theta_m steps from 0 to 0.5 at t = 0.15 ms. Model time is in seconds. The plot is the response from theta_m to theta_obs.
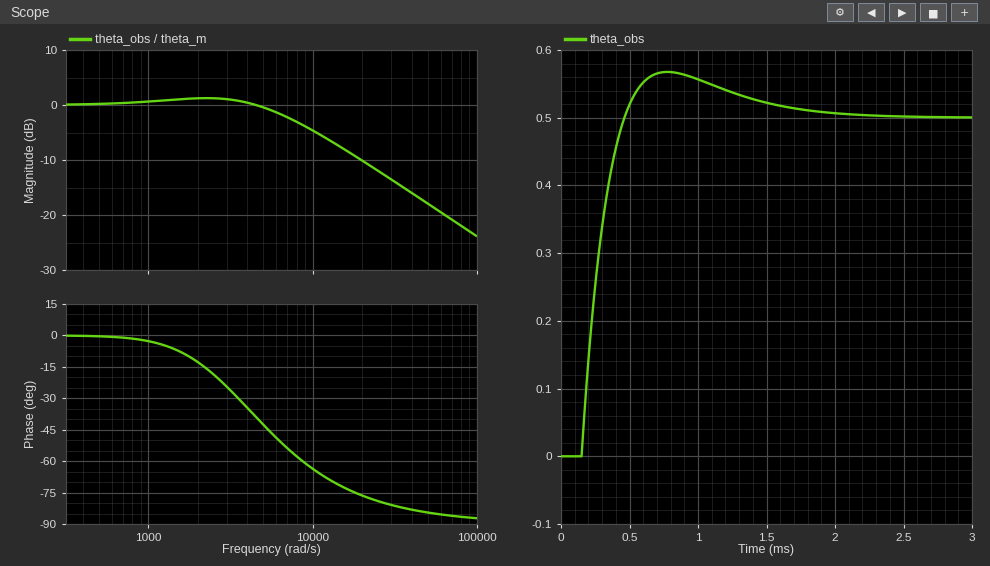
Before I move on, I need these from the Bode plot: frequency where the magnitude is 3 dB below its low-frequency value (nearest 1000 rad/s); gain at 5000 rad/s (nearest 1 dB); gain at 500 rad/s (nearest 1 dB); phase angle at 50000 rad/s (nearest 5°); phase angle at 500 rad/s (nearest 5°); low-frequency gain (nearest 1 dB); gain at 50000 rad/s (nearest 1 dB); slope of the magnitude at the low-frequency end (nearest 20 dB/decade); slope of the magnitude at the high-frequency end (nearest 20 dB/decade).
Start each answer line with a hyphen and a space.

- 8000 rad/s
- 0 dB
- 0 dB
- -85°
- 0°
- 0 dB
- -18 dB
- 0 dB/decade
- -20 dB/decade
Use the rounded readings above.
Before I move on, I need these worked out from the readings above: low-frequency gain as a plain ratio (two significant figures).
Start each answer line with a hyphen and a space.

- 1.0
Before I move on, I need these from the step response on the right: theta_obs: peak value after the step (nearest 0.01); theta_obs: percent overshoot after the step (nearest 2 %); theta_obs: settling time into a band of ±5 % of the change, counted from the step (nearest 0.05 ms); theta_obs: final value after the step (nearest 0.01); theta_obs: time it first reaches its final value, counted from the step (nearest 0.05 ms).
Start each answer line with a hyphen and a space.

- 0.57
- 14 %
- 1.30 ms
- 0.50
- 0.30 ms
